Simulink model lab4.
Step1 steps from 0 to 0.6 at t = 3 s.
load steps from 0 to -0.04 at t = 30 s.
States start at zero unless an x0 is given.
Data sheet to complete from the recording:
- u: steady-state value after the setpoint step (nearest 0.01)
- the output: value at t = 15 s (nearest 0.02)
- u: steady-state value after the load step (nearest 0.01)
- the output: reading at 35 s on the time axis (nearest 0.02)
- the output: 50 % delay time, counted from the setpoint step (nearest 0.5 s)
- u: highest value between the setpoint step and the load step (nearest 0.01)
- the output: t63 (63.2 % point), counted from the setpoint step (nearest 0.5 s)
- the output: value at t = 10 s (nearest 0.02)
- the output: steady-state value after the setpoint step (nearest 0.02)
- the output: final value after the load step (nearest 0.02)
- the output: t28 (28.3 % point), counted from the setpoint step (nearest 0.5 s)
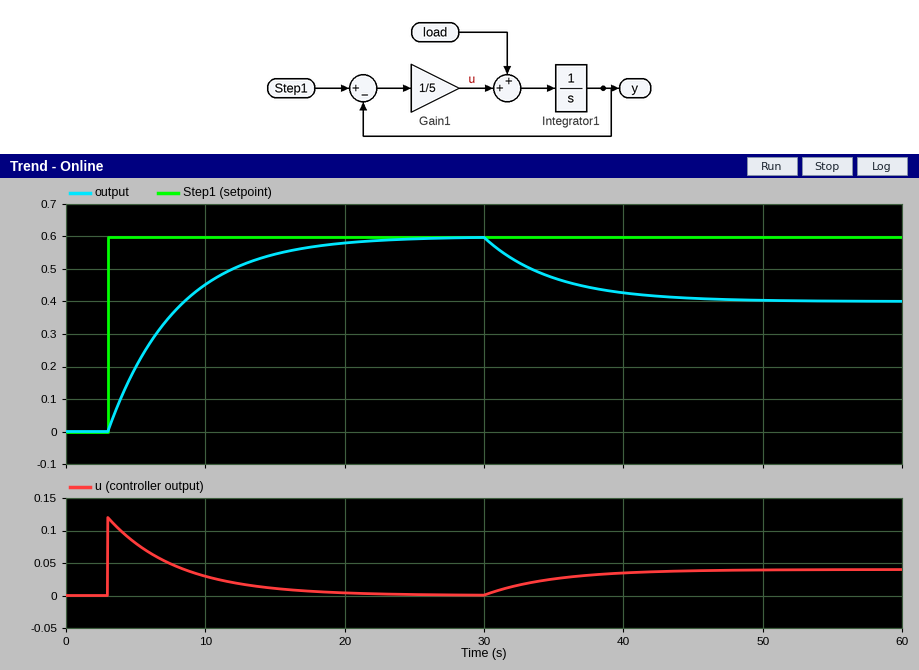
0.00
0.54
0.04
0.48
3.5 s
0.12
5.0 s
0.46
0.60
0.40
1.5 s
